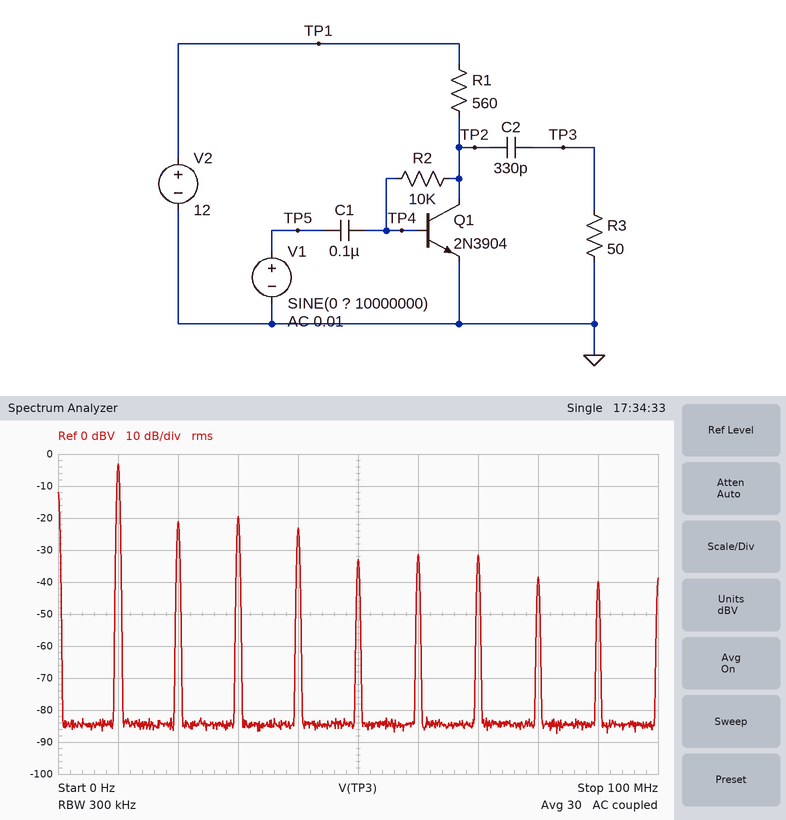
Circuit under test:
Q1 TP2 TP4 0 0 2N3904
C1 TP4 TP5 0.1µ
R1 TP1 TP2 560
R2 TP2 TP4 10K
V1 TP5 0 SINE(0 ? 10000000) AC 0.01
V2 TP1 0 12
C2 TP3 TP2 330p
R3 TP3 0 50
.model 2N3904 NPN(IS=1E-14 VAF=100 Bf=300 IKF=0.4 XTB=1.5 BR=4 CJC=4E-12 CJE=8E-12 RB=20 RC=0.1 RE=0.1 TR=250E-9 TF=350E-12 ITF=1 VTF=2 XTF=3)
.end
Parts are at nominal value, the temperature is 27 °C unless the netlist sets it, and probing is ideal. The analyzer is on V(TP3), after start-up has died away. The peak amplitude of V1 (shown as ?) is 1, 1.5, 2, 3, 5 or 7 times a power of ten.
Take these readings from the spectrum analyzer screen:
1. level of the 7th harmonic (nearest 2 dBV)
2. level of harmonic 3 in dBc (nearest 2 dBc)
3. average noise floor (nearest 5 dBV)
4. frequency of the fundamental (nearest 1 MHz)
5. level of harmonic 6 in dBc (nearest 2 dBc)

-32 dBV
-16 dBc
-85 dBV
10 MHz
-28 dBc
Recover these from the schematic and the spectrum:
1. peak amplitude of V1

70 mV
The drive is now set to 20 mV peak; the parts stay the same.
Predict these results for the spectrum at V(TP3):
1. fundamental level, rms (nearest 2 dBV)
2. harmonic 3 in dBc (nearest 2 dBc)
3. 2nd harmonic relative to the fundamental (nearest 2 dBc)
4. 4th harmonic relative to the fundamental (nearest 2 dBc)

-10 dBV
-42 dBc
-22 dBc
-54 dBc
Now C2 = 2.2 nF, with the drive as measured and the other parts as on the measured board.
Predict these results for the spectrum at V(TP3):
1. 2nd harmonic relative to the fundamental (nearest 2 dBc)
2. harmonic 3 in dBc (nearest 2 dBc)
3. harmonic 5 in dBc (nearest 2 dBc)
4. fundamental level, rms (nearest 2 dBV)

-12 dBc
-20 dBc
-26 dBc
-2 dBV
